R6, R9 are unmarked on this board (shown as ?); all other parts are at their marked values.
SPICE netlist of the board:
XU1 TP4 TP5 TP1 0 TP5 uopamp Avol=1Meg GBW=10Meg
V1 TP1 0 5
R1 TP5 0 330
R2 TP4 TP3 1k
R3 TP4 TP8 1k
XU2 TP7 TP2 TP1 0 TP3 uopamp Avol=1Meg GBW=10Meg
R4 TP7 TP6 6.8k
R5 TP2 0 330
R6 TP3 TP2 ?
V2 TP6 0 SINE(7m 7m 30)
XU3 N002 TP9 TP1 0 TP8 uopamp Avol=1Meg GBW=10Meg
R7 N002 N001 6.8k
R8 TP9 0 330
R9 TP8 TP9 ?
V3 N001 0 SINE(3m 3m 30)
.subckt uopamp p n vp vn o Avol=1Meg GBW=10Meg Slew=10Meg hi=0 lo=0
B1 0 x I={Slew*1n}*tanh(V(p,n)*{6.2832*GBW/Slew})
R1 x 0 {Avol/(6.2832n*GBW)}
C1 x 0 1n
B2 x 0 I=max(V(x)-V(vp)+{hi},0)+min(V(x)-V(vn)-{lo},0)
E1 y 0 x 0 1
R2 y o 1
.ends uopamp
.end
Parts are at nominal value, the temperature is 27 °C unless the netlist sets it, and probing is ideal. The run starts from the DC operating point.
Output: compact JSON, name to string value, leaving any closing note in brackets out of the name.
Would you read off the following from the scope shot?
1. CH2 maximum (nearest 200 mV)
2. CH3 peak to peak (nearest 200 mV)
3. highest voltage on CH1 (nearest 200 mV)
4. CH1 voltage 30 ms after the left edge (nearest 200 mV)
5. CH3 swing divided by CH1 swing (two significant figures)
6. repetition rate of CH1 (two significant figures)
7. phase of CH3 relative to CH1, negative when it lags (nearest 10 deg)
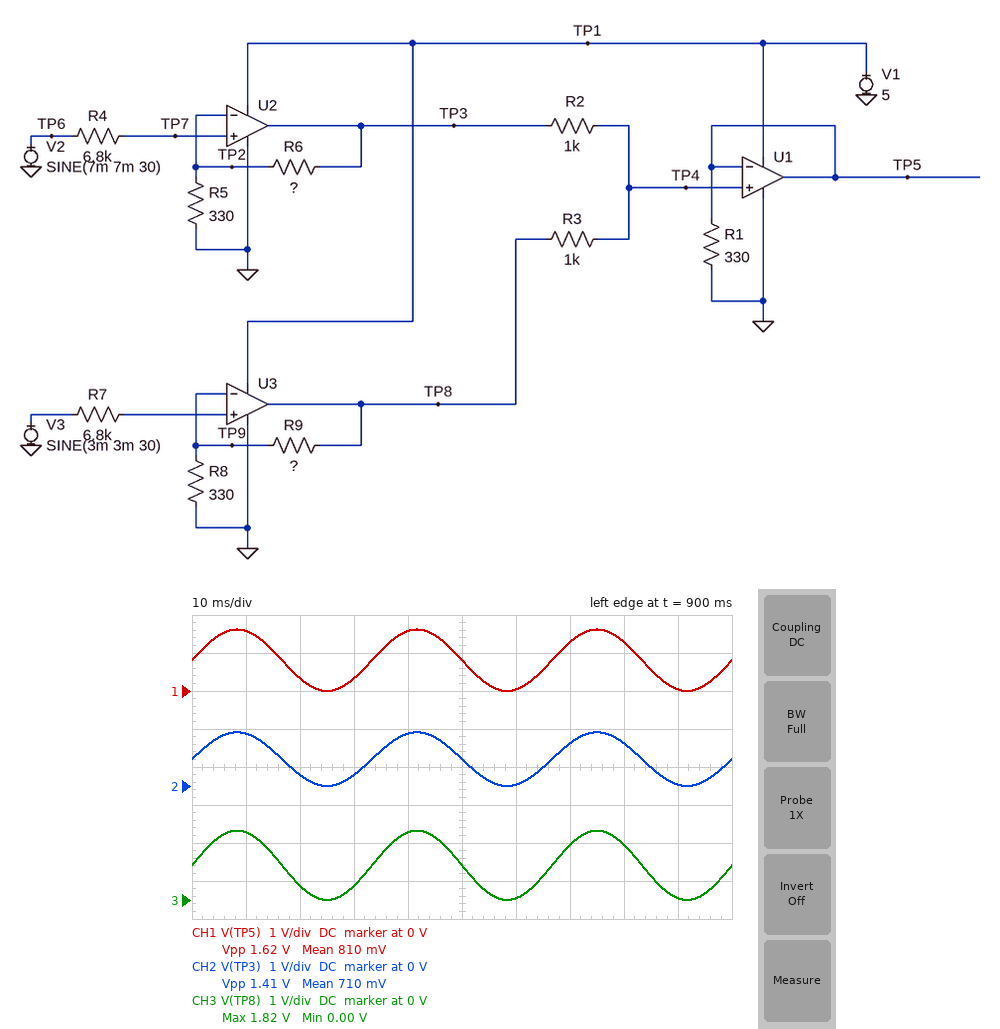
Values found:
{"CH2 maximum": "1.4 V", "CH3 peak to peak": "1.8 V", "highest voltage on CH1": "1.6 V", "CH1 voltage 30 ms after the left edge": "400 mV", "CH3 swing divided by CH1 swing": "1.1", "repetition rate of CH1": "30 Hz", "phase of CH3 relative to CH1, negative when it lags": "0 deg"}
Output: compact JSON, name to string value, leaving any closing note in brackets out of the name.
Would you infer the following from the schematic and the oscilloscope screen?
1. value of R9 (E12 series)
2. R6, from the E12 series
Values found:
{"value of R9": "100 kΩ", "R6, from the E12 series": "33 kΩ"}
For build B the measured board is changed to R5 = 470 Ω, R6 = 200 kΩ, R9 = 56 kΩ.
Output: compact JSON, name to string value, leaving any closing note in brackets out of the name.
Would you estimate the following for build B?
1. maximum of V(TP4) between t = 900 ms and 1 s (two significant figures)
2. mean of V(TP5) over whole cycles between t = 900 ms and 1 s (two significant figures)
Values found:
{"maximum of V(TP4) between t = 900 ms and 1 s": "3.0 V", "mean of V(TP5) over whole cycles between t = 900 ms and 1 s": "1.7 V"}
